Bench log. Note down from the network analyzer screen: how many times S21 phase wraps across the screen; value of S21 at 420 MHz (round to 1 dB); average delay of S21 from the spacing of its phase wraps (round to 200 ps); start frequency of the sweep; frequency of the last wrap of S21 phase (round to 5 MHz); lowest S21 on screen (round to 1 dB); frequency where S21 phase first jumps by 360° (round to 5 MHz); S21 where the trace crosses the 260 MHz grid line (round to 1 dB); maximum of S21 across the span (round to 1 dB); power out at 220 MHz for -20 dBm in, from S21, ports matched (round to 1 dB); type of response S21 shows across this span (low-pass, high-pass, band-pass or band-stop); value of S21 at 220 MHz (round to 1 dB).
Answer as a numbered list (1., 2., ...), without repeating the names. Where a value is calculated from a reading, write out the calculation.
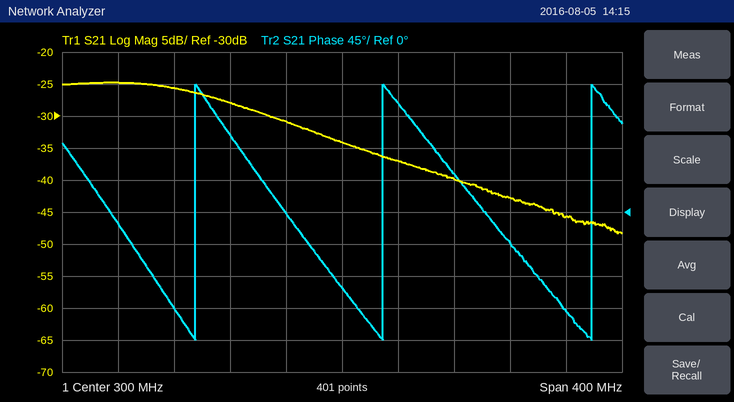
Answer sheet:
1. 3
2. -43 dB
3. 2 cycles / (480 MHz − 195 MHz) ≈ 7.0 ns
4. 100 MHz
5. 480 MHz
6. -48 dB
7. 195 MHz
8. -31 dB
9. -25 dB
10. -20 dBm + (-28 dB) = -48 dBm
11. low-pass
12. -28 dB
